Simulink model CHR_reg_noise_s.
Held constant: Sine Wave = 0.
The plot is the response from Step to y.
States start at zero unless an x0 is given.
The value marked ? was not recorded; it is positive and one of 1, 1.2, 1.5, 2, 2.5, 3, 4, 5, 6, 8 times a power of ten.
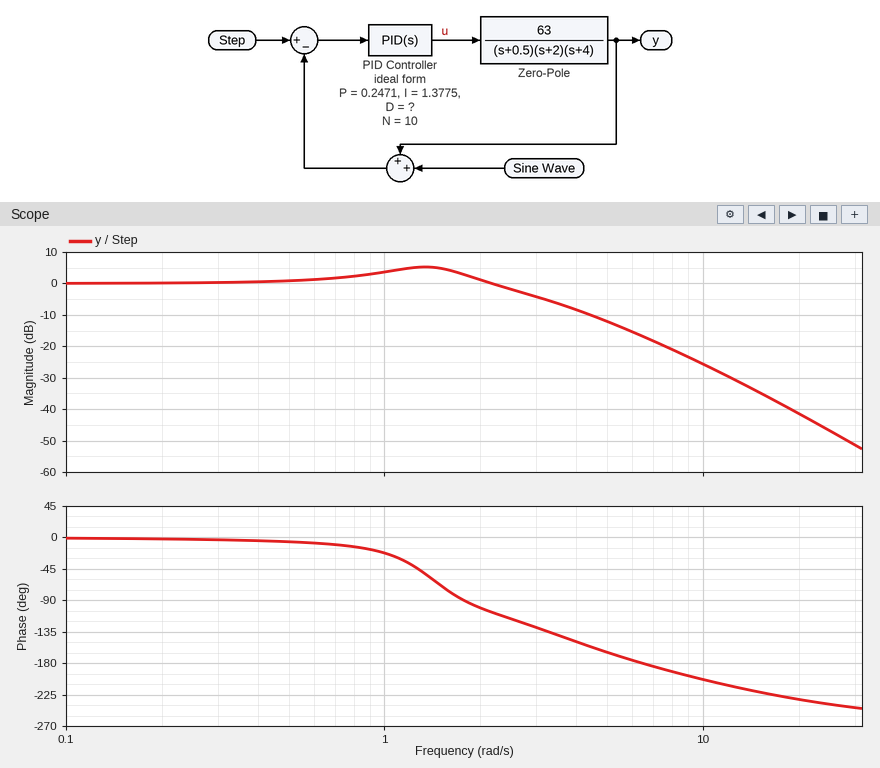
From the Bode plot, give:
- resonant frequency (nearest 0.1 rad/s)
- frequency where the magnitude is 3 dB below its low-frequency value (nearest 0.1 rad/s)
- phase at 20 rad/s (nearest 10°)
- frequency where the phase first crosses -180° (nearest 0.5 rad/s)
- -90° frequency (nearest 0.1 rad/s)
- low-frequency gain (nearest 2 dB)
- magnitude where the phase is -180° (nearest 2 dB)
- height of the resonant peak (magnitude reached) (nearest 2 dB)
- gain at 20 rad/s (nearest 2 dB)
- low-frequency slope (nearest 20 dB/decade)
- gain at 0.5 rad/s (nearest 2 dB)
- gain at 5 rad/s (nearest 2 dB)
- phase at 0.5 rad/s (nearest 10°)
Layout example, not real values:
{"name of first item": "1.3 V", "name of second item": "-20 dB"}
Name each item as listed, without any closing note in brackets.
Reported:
{"resonant frequency": "1.3 rad/s", "frequency where the magnitude is 3 dB below its low-frequency value": "2.7 rad/s", "phase at 20 rad/s": "-230°", "frequency where the phase first crosses -180°": "6.5 rad/s", "-90° frequency": "1.8 rad/s", "low-frequency gain": "0 dB", "magnitude where the phase is -180°": "-16 dB", "height of the resonant peak (magnitude reached)": "6 dB", "gain at 20 rad/s": "-42 dB", "low-frequency slope": "0 dB/decade", "gain at 0.5 rad/s": "0 dB", "gain at 5 rad/s": "-12 dB", "phase at 0.5 rad/s": "-10°"}
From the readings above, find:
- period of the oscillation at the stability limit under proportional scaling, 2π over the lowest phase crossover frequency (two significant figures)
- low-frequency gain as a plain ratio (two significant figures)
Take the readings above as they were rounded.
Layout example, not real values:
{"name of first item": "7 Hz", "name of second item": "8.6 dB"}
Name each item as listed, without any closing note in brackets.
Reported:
{"period of the oscillation at the stability limit under proportional scaling, 2π over the lowest phase crossover frequency": "0.97 s", "low-frequency gain as a plain ratio": "1.0"}
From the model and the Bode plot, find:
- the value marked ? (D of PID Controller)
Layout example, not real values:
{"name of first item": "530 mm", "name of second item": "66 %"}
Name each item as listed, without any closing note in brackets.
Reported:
{"the value marked ?": "0.4"}
